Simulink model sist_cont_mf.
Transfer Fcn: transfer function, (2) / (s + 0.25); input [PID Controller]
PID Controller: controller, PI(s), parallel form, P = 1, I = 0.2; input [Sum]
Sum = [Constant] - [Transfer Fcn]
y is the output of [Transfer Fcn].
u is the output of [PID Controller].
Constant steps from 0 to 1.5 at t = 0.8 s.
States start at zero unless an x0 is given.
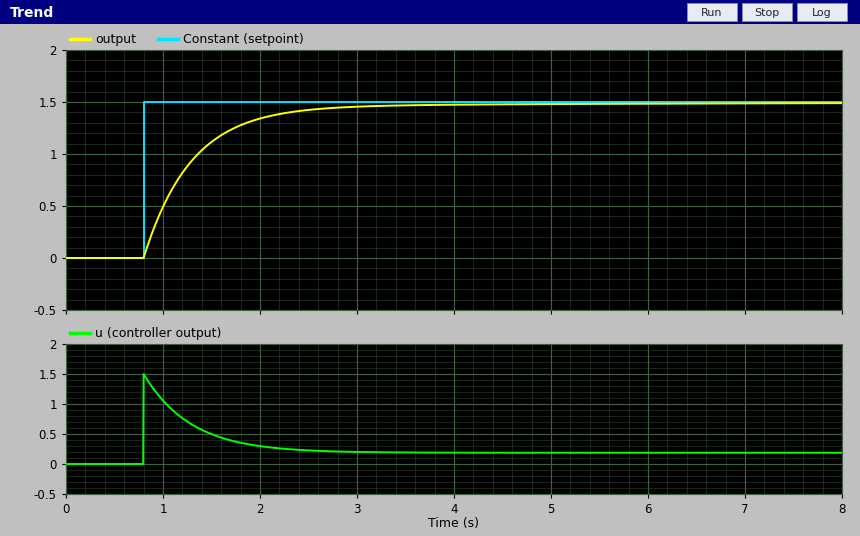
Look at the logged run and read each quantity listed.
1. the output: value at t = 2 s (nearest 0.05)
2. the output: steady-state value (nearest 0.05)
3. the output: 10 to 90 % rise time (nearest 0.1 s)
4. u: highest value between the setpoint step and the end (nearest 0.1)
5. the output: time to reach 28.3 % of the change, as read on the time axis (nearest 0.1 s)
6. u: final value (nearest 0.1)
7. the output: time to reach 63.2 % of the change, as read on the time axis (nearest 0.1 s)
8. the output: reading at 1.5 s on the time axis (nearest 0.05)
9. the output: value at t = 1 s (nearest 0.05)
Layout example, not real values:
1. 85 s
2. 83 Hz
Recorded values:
1. 1.35
2. 1.50
3. 1.2 s
4. 1.5
5. 1.0 s
6. 0.2
7. 1.3 s
8. 1.10
9. 0.50
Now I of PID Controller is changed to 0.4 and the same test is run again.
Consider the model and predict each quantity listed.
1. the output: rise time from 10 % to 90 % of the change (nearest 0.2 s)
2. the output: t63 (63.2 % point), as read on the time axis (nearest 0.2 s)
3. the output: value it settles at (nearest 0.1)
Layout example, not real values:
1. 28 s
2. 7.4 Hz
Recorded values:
1. 1.0 s
2. 1.2 s
3. 1.5
